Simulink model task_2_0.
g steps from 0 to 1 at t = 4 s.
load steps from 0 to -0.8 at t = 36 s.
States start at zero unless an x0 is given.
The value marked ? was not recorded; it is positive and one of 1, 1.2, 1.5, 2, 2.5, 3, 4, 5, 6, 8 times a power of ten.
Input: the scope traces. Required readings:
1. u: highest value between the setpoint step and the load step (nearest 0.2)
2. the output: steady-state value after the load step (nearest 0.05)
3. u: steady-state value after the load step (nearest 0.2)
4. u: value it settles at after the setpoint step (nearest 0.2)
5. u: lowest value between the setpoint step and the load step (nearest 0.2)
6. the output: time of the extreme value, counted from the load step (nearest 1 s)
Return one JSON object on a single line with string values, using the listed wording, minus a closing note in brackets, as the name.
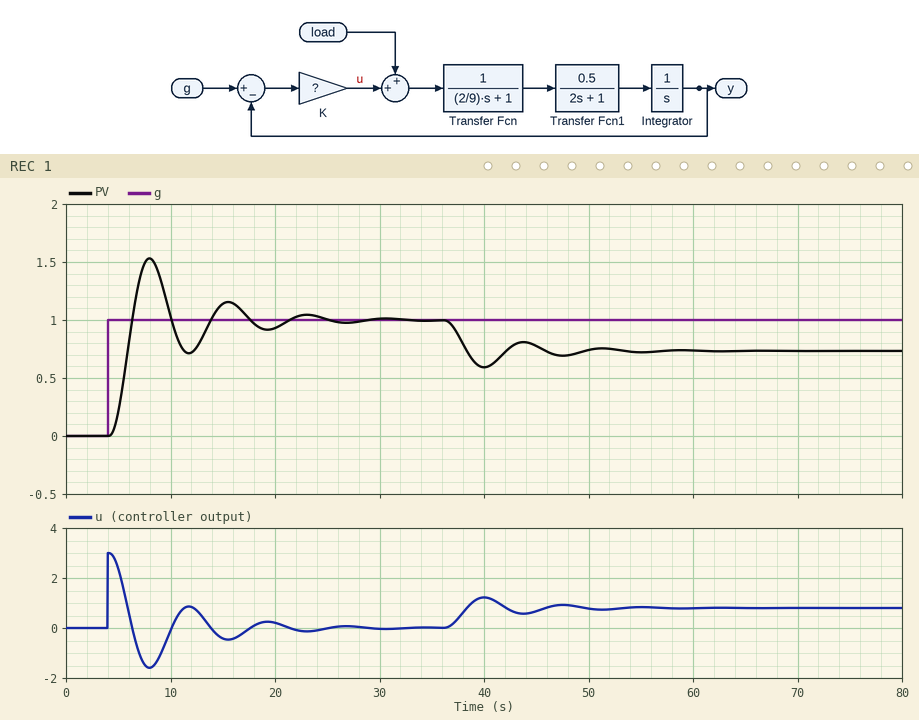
{"u: highest value between the setpoint step and the load step": "3.0", "the output: steady-state value after the load step": "0.75", "u: steady-state value after the load step": "0.8", "u: value it settles at after the setpoint step": "0.0", "u: lowest value between the setpoint step and the load step": "-1.6", "the output: time of the extreme value, counted from the load step": "4 s"}
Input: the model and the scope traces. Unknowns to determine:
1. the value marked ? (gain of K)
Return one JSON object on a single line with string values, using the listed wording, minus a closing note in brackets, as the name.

{"the value marked ?": "3"}
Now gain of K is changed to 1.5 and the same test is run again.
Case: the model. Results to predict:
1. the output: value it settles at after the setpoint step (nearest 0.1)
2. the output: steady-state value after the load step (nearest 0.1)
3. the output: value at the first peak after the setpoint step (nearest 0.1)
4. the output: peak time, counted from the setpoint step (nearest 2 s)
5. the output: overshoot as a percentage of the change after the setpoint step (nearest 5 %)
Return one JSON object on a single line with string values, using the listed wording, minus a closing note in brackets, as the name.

{"the output: value it settles at after the setpoint step": "1.0", "the output: steady-state value after the load step": "0.5", "the output: value at the first peak after the setpoint step": "1.3", "the output: peak time, counted from the setpoint step": "6 s", "the output: overshoot as a percentage of the change after the setpoint step": "30 %"}
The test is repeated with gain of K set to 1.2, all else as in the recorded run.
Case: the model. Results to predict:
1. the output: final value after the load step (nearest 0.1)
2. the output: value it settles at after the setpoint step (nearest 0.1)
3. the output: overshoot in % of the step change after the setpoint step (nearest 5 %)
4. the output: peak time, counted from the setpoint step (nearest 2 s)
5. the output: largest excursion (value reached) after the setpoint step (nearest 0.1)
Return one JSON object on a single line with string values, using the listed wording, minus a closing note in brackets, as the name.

{"the output: final value after the load step": "0.3", "the output: value it settles at after the setpoint step": "1.0", "the output: overshoot in % of the step change after the setpoint step": "25 %", "the output: peak time, counted from the setpoint step": "6 s", "the output: largest excursion (value reached) after the setpoint step": "1.3"}
